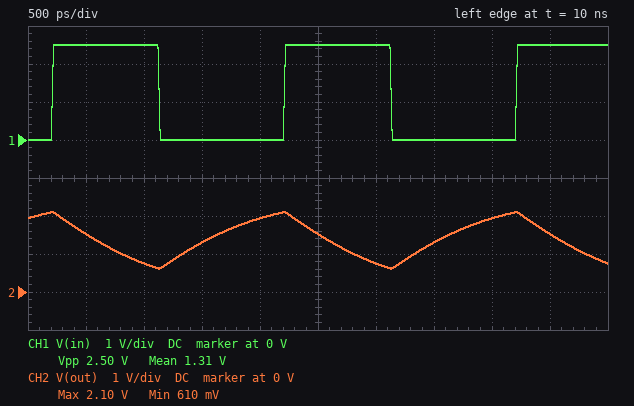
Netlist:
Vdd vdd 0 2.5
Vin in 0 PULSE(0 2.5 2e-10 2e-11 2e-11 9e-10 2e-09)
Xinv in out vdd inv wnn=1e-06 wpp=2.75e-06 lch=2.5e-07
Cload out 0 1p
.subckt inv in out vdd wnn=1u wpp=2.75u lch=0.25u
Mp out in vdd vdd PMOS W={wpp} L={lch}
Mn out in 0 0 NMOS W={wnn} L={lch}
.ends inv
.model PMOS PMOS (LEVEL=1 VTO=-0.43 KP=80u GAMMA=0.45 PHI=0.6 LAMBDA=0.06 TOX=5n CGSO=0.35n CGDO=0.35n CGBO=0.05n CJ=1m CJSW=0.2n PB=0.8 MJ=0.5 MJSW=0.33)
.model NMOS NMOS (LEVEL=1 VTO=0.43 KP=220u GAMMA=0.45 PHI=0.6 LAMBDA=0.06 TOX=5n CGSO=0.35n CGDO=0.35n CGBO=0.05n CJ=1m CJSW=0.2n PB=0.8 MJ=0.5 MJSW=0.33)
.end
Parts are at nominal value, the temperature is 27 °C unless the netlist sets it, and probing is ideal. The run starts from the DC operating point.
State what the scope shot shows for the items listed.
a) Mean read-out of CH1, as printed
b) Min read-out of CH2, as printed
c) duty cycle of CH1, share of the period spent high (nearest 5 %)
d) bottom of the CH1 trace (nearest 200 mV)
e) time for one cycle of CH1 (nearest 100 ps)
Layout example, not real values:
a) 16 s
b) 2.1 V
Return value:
a) 1.31 V
b) 610 mV
c) 45 %
d) 0 V
e) 2.0 ns
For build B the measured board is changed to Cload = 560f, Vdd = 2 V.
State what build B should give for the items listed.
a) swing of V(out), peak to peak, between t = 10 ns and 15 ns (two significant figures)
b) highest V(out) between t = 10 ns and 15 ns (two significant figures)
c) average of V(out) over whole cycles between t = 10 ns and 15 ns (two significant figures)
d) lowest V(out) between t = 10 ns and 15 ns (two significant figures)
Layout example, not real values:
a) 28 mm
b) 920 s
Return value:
a) 1.6 V
b) 1.7 V
c) 900 mV
d) 130 mV
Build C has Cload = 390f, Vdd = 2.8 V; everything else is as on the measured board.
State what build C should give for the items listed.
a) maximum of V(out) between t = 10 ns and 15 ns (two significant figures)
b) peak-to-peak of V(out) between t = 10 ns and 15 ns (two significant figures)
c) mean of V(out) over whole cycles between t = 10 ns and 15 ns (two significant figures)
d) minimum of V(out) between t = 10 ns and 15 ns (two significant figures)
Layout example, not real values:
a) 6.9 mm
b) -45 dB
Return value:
a) 2.8 V
b) 2.7 V
c) 1.6 V
d) 90 mV
